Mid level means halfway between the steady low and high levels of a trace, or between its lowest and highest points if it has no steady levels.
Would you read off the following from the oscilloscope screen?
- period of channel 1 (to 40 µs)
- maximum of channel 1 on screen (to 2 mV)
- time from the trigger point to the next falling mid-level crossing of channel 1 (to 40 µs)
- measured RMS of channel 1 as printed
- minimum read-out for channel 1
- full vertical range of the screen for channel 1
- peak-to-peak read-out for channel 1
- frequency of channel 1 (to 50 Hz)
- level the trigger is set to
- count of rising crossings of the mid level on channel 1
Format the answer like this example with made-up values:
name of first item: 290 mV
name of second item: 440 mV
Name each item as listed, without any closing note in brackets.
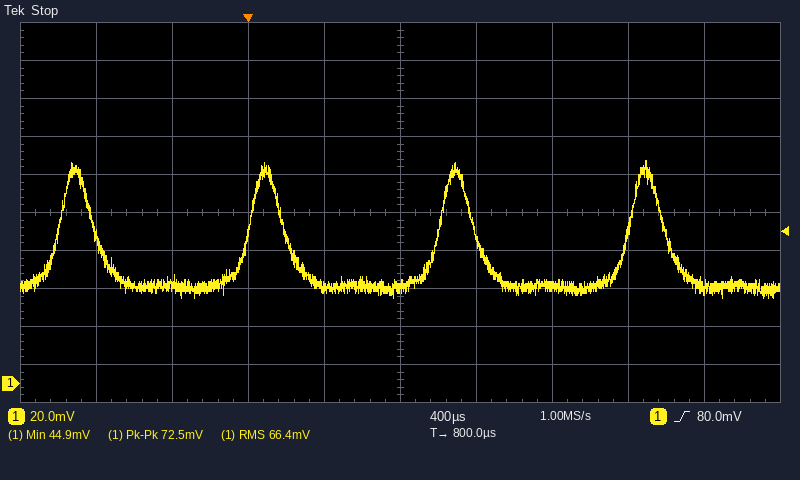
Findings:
period of channel 1: 1.00 ms
maximum of channel 1 on screen: 118 mV
time from the trigger point to the next falling mid-level crossing of channel 1: 200 µs
measured RMS of channel 1 as printed: 66.4 mV
minimum read-out for channel 1: 44.9 mV
full vertical range of the screen for channel 1: 200 mV
peak-to-peak read-out for channel 1: 72.5 mV
frequency of channel 1: 1.00 kHz
level the trigger is set to: 80.0 mV
count of rising crossings of the mid level on channel 1: 4
